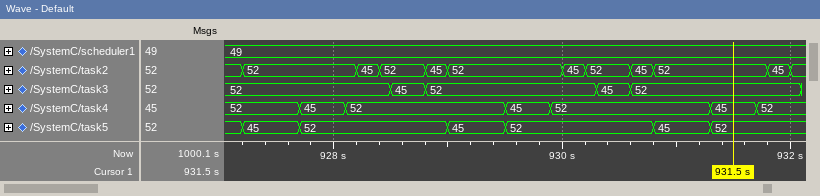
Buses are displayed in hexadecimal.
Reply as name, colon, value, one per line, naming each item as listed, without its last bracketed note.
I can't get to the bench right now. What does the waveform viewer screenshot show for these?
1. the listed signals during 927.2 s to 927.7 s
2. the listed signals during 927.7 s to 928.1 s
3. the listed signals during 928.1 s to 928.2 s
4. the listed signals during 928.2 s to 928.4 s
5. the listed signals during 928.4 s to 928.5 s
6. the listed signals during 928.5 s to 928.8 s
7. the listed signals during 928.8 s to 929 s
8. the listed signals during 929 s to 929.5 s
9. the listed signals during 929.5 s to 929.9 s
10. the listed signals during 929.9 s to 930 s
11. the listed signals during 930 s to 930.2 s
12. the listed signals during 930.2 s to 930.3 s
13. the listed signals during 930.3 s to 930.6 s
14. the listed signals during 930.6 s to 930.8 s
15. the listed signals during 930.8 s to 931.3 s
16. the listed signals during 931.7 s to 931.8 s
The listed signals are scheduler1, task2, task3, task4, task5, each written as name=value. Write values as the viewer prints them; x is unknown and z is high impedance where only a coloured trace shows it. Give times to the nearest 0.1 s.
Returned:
the listed signals during 927.2 s to 927.7 s: scheduler1=49, task2=52, task3=52, task4=52, task5=45
the listed signals during 927.7 s to 928.1 s: scheduler1=49, task2=52, task3=52, task4=45, task5=52
the listed signals during 928.1 s to 928.2 s: scheduler1=49, task2=52, task3=52, task4=52, task5=52
the listed signals during 928.2 s to 928.4 s: scheduler1=49, task2=45, task3=52, task4=52, task5=52
the listed signals during 928.4 s to 928.5 s: scheduler1=49, task2=52, task3=52, task4=52, task5=52
the listed signals during 928.5 s to 928.8 s: scheduler1=49, task2=52, task3=45, task4=52, task5=52
the listed signals during 928.8 s to 929 s: scheduler1=49, task2=45, task3=52, task4=52, task5=52
the listed signals during 929 s to 929.5 s: scheduler1=49, task2=52, task3=52, task4=52, task5=45
the listed signals during 929.5 s to 929.9 s: scheduler1=49, task2=52, task3=52, task4=45, task5=52
the listed signals during 929.9 s to 930 s: scheduler1=49, task2=52, task3=52, task4=52, task5=52
the listed signals during 930 s to 930.2 s: scheduler1=49, task2=45, task3=52, task4=52, task5=52
the listed signals during 930.2 s to 930.3 s: scheduler1=49, task2=52, task3=52, task4=52, task5=52
the listed signals during 930.3 s to 930.6 s: scheduler1=49, task2=52, task3=45, task4=52, task5=52
the listed signals during 930.6 s to 930.8 s: scheduler1=49, task2=45, task3=52, task4=52, task5=52
the listed signals during 930.8 s to 931.3 s: scheduler1=49, task2=52, task3=52, task4=52, task5=45
the listed signals during 931.7 s to 931.8 s: scheduler1=49, task2=52, task3=52, task4=52, task5=52
